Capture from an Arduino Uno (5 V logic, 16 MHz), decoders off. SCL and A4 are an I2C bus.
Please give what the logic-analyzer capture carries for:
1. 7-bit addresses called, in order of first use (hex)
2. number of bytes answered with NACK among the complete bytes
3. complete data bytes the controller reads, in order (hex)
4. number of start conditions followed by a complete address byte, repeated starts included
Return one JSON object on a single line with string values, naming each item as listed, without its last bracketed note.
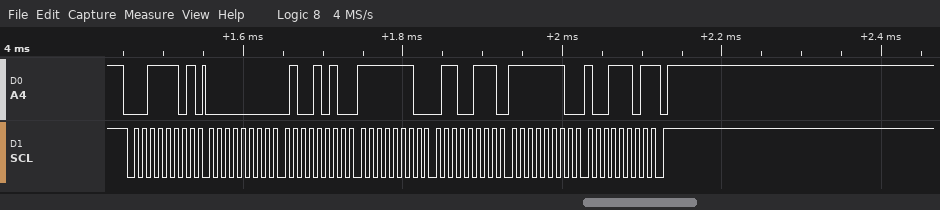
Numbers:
{"7-bit addresses called, in order of first use": "0x1E", "number of bytes answered with NACK among the complete bytes": "1", "complete data bytes the controller reads, in order": "00 4A FE 67 FE 9D", "number of start conditions followed by a complete address byte, repeated starts included": "1"}
